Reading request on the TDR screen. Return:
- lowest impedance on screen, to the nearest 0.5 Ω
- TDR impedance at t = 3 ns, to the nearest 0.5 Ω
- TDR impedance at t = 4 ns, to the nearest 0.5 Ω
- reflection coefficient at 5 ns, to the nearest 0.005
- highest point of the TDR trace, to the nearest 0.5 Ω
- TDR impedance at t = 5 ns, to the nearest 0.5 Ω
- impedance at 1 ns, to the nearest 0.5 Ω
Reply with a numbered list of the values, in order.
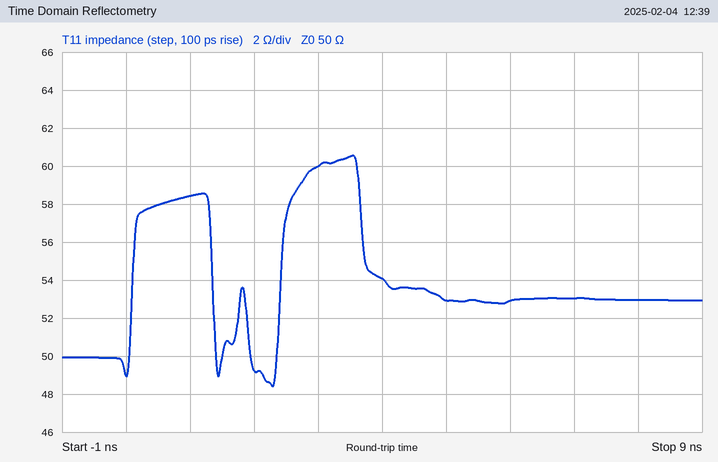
1. 48.5 Ω
2. 60.0 Ω
3. 54.0 Ω
4. +0.030
5. 60.5 Ω
6. 53.0 Ω
7. 58.5 Ω
